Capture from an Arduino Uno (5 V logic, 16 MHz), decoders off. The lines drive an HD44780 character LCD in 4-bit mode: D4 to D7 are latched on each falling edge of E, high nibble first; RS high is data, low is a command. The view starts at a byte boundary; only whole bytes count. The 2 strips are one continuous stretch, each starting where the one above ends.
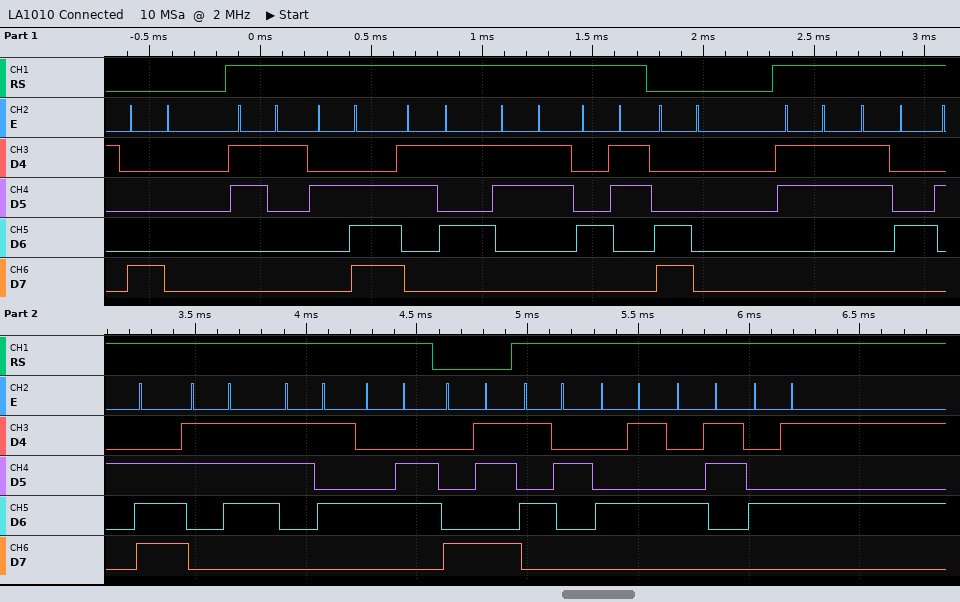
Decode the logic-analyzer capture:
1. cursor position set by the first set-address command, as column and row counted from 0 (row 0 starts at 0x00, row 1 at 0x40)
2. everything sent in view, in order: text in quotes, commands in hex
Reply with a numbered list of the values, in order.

1. column 0, row 0
2. 0x80 "1.53C" 0xC0 "34.75F" 0x8B "RECE"
